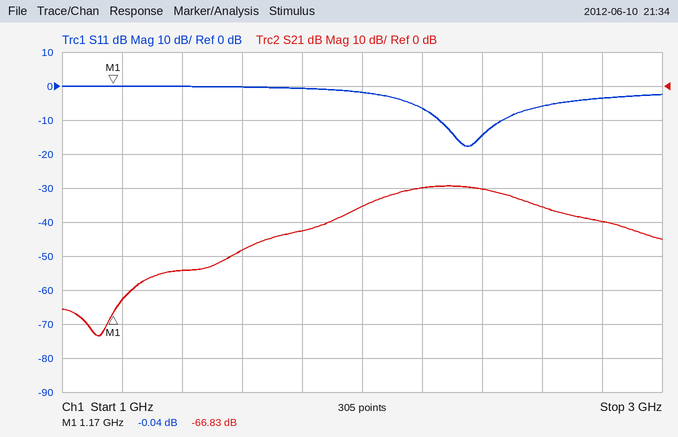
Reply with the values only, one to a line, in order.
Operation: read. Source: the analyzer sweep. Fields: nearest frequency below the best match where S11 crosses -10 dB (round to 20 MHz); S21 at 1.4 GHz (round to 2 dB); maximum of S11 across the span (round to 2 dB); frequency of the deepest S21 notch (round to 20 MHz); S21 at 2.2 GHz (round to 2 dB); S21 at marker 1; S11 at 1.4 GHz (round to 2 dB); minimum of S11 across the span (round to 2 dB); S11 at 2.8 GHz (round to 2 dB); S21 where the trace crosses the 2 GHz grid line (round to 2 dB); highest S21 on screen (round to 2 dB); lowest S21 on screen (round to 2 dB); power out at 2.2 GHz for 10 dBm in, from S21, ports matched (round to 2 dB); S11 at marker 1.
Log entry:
2.26 GHz
-54 dB
0 dB
1.12 GHz
-30 dB
-66.83 dB
0 dB
-18 dB
-4 dB
-36 dB
-30 dB
-74 dB
-20 dBm
-0.04 dB
